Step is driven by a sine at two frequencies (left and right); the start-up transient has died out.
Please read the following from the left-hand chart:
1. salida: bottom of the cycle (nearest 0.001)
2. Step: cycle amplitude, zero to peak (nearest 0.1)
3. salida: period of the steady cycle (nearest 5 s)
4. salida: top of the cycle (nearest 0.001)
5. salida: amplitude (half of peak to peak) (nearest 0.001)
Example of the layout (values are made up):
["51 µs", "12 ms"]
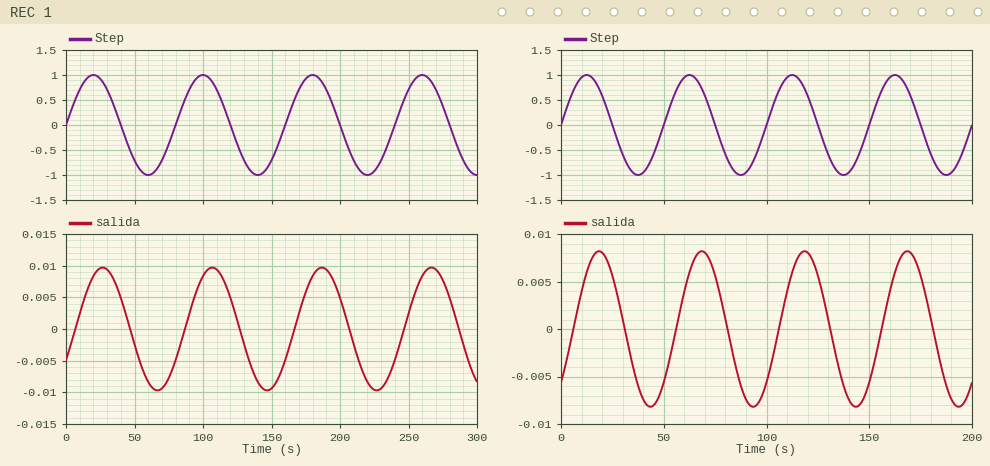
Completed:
["-0.010", "1.0", "80 s", "0.010", "0.010"]
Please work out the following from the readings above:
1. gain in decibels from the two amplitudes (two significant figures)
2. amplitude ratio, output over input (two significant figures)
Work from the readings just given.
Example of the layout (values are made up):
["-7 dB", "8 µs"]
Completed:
["-40 dB", "0.010"]
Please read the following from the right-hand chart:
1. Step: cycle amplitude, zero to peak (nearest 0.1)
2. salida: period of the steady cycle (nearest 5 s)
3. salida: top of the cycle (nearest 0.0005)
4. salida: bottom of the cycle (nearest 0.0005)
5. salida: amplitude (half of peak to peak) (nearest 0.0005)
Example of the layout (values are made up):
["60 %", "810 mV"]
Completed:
["1.0", "50 s", "0.0080", "-0.0080", "0.0080"]
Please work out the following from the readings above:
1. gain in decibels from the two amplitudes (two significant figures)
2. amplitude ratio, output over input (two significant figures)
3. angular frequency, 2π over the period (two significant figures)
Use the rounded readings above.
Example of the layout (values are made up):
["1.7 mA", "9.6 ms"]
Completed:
["-42 dB", "0.0080", "0.13 rad/s"]
